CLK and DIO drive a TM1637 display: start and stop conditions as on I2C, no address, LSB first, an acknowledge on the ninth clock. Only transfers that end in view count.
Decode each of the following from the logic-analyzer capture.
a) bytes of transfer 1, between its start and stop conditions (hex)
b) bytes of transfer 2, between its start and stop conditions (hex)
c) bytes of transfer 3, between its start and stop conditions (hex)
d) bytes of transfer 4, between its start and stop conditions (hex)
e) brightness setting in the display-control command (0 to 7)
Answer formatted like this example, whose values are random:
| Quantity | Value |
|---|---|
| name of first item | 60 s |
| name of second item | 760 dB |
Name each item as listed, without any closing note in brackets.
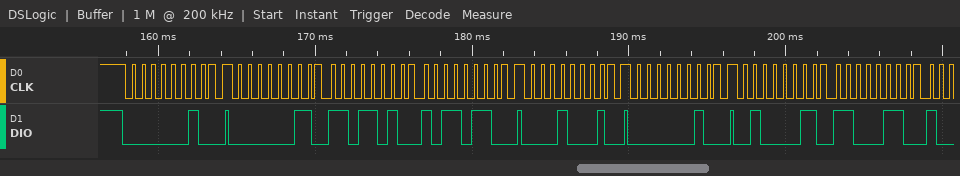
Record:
| Quantity | Value |
|---|---|
| bytes of transfer 1, between its start and stop conditions | 40 |
| bytes of transfer 2, between its start and stop conditions | C0 5B 6D |
| bytes of transfer 3, between its start and stop conditions | 88 |
| bytes of transfer 4, between its start and stop conditions | 40 |
| brightness setting in the display-control command | 0 |
